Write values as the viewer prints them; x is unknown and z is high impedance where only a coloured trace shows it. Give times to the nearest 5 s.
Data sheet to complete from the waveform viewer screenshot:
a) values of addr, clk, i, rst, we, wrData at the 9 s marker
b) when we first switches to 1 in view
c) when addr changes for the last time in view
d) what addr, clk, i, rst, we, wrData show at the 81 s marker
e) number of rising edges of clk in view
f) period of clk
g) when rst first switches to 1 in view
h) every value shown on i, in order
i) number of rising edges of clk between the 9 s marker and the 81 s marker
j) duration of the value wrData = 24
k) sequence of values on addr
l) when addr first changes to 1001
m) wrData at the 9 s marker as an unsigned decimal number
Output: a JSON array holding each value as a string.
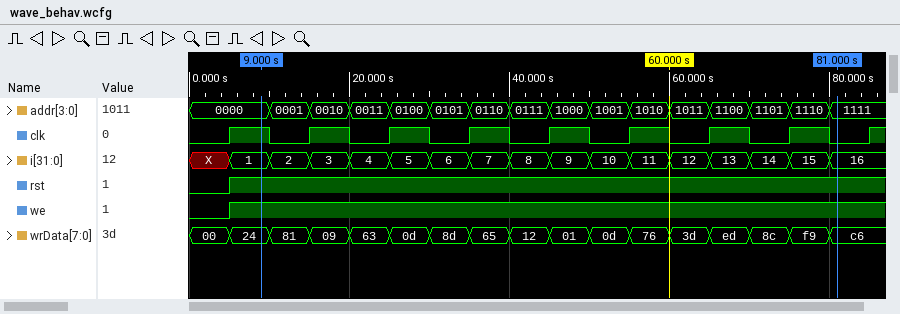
["addr=0000, clk=1, i=1, rst=1, we=1, wrData=24", "5 s", "80 s", "addr=1111, clk=0, i=16, rst=1, we=1, wrData=c6", "9", "10 s", "5 s", "X, 1, 2, 3, 4, 5, 6, 7, 8, 9, 10, 11, 12, 13, 14, 15, 16", "7", "5 s", "0000, 0001, 0010, 0011, 0100, 0101, 0110, 0111, 1000, 1001, 1010, 1011, 1100, 1101, 1110, 1111", "50 s", "36"]
